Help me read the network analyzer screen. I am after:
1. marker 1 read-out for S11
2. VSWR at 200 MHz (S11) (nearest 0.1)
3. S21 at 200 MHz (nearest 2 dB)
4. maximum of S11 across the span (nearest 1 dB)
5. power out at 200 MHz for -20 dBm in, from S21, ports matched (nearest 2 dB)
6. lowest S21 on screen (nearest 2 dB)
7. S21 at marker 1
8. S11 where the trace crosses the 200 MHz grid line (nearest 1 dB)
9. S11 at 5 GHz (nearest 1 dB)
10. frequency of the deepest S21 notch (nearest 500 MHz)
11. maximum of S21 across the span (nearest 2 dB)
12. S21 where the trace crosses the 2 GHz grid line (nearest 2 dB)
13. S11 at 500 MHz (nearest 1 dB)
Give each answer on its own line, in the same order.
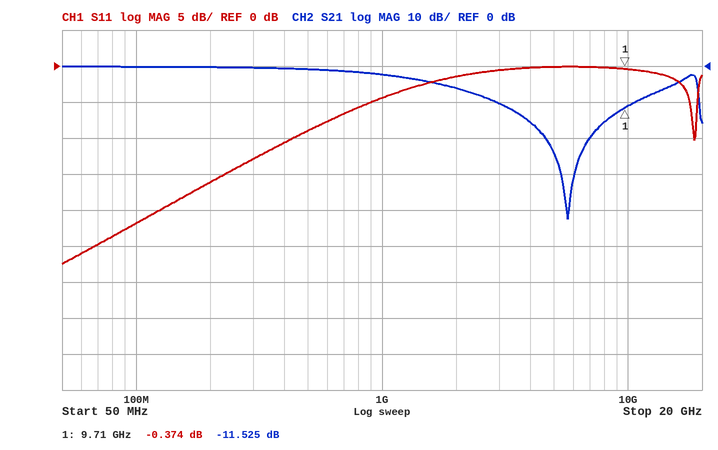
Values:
-0.374 dB
1.4
0 dB
0 dB
-20 dBm
-42 dB
-11.525 dB
-16 dB
0 dB
5.5 GHz
0 dB
-6 dB
-9 dB
